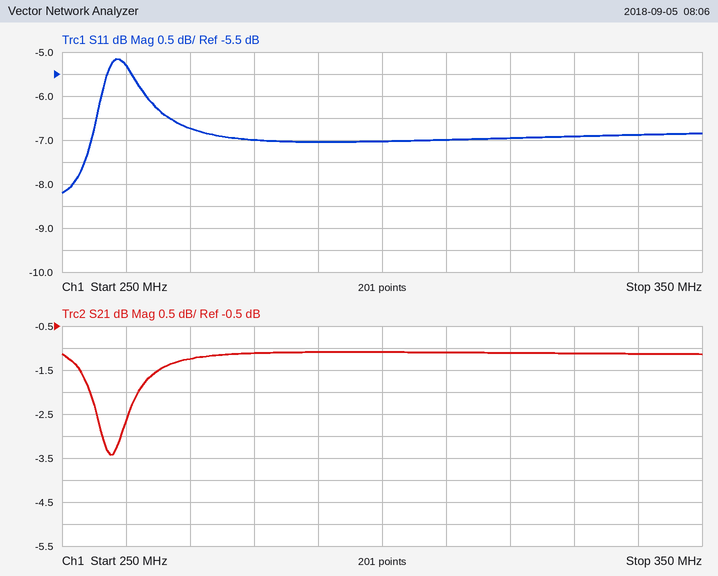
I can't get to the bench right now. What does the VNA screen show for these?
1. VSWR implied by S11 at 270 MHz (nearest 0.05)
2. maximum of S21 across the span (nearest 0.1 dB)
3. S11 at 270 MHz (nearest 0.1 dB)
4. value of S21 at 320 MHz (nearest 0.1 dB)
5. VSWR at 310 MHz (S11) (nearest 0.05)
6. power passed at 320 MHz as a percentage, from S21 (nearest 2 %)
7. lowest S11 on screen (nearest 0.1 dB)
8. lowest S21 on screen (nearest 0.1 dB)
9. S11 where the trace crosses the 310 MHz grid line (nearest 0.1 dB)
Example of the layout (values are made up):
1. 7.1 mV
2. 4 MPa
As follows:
1. 2.70
2. -1.1 dB
3. -6.7 dB
4. -1.1 dB
5. 2.60
6. 78 %
7. -8.2 dB
8. -3.4 dB
9. -7.0 dB
